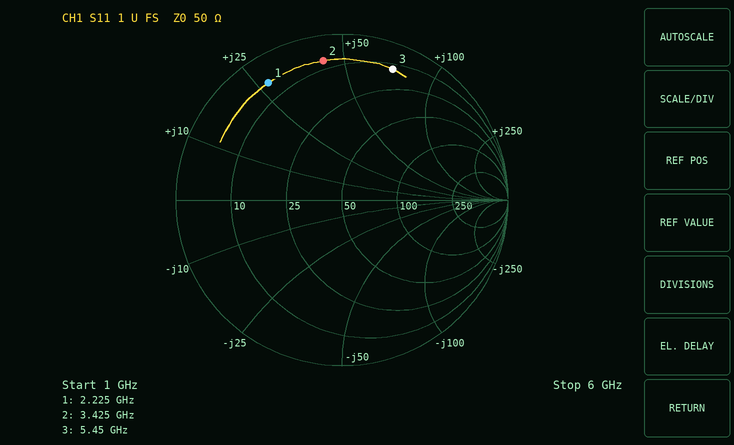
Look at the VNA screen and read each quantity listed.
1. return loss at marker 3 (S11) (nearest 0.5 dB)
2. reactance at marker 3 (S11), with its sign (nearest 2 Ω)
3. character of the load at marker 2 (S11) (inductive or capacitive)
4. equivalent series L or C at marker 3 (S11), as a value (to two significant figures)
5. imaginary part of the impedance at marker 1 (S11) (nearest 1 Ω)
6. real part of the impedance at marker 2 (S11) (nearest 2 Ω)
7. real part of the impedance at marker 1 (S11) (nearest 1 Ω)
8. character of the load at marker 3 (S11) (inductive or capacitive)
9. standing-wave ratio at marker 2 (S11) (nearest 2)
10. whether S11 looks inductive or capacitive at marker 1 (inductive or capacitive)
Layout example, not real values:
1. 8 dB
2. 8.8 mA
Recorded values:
1. 1.5 dB
2. +72 Ω
3. inductive
4. 2.1 nH
5. +27 Ω
6. 8 Ω
7. 6 Ω
8. inductive
9. 12
10. inductive
